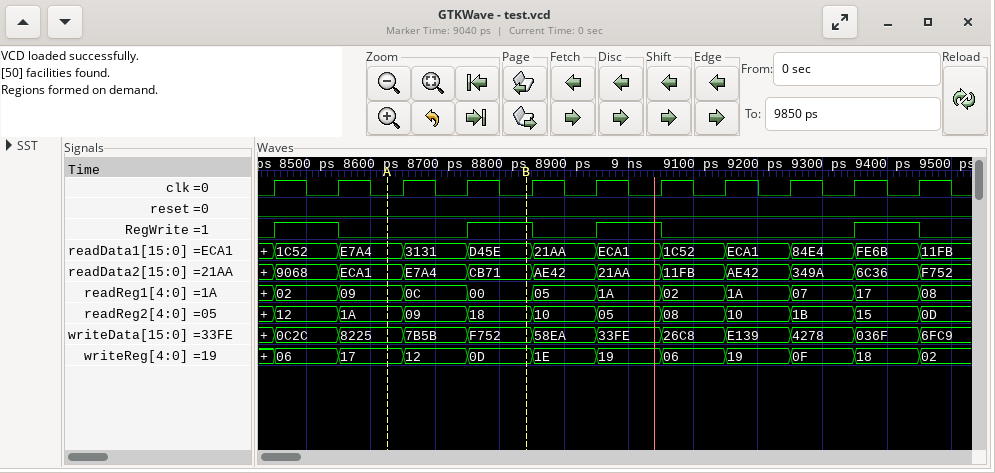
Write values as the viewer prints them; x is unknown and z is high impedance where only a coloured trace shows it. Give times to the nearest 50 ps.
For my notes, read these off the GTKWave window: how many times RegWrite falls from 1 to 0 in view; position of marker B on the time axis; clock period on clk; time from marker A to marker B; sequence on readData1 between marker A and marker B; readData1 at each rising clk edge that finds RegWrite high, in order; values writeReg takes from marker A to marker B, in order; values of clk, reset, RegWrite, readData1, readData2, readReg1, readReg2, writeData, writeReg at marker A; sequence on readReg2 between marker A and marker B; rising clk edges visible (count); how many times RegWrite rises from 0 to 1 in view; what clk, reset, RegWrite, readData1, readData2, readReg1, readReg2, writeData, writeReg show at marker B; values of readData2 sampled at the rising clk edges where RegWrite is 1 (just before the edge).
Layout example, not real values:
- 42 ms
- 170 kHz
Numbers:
- 4
- 8850 ps
- 100 ps
- 200 ps
- E7A4, 3131, D45E
- 1C52, D45E, ECA1, FE6B
- 17, 12, 0D
- clk=0, reset=0, RegWrite=0, readData1=E7A4, readData2=ECA1, readReg1=09, readReg2=1A, writeData=8225, writeReg=17
- 1A, 09, 18
- 11
- 4
- clk=0, reset=0, RegWrite=1, readData1=D45E, readData2=CB71, readReg1=00, readReg2=18, writeData=F752, writeReg=0D
- 9068, CB71, 21AA, 6C36
